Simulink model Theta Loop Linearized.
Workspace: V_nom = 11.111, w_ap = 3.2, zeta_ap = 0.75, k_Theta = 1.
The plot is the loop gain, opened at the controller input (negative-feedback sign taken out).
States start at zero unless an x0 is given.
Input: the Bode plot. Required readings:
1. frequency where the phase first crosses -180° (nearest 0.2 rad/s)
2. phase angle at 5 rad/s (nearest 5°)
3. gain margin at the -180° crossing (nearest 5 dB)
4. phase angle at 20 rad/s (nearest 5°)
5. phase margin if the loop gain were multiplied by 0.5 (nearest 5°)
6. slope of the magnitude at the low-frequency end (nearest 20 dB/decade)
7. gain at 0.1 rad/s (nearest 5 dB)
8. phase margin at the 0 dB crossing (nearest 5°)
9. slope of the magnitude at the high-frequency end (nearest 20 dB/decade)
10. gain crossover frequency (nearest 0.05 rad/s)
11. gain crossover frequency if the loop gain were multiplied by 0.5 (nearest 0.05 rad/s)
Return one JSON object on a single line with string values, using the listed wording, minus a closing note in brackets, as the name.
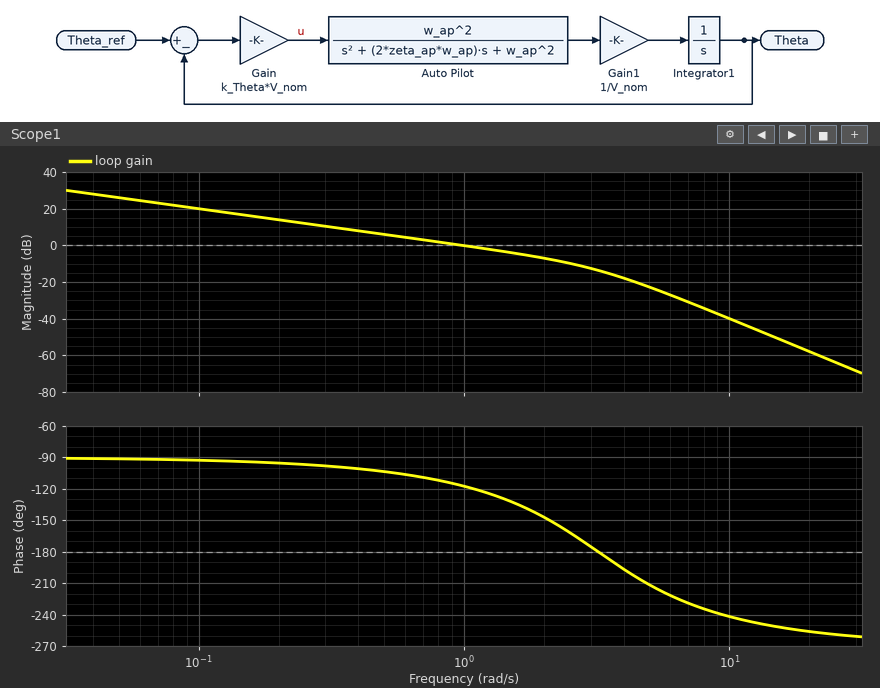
{"frequency where the phase first crosses -180°": "3.2 rad/s", "phase angle at 5 rad/s": "-210°", "gain margin at the -180° crossing": "15 dB", "phase angle at 20 rad/s": "-255°", "phase margin if the loop gain were multiplied by 0.5": "75°", "slope of the magnitude at the low-frequency end": "-20 dB/decade", "gain at 0.1 rad/s": "20 dB", "phase margin at the 0 dB crossing": "65°", "slope of the magnitude at the high-frequency end": "-60 dB/decade", "gain crossover frequency": "1.00 rad/s", "gain crossover frequency if the loop gain were multiplied by 0.5": "0.50 rad/s"}
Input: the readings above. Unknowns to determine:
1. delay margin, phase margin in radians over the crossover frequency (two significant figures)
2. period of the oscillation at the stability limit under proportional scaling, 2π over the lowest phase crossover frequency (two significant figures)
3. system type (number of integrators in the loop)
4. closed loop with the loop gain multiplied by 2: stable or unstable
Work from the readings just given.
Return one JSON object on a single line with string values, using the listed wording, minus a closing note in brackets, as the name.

{"delay margin, phase margin in radians over the crossover frequency": "1.1 s", "period of the oscillation at the stability limit under proportional scaling, 2π over the lowest phase crossover frequency": "2.0 s", "system type": "1", "closed loop with the loop gain multiplied by 2: stable or unstable": "stable"}
